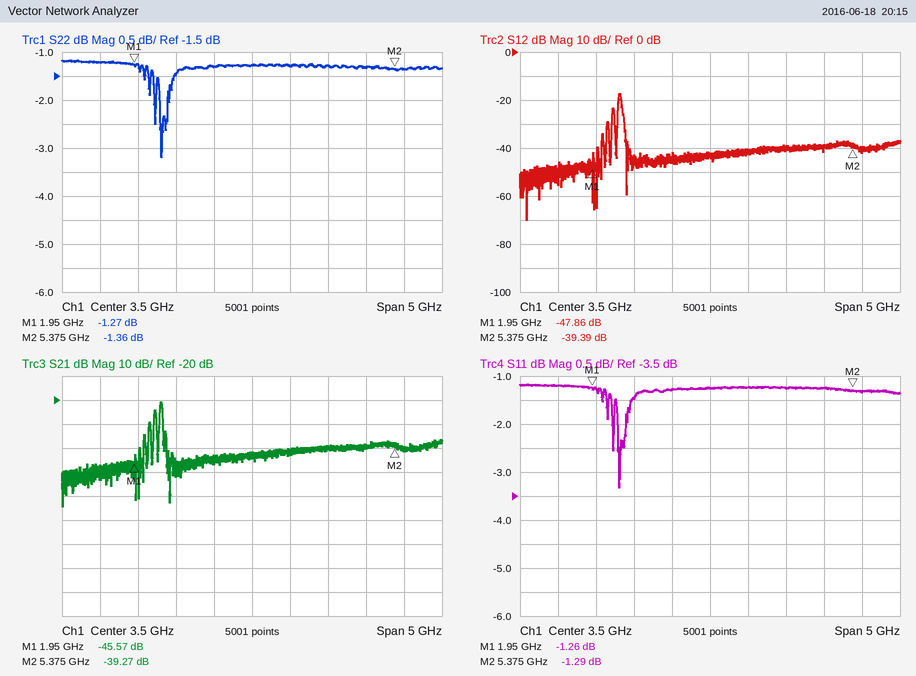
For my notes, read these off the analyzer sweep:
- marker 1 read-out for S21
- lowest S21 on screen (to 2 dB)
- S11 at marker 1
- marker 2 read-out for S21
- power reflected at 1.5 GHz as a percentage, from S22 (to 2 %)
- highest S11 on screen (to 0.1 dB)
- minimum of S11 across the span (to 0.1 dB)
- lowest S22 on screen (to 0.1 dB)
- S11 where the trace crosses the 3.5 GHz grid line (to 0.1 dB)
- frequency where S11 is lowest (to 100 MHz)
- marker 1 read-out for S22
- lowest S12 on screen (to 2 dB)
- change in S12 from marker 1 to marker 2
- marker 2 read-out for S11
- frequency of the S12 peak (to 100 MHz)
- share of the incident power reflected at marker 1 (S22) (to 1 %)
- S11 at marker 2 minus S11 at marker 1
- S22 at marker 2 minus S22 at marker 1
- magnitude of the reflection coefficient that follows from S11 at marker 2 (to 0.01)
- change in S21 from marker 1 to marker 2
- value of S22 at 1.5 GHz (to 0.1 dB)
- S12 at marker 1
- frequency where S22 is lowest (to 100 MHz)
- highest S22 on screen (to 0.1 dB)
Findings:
-45.57 dB
-64 dB
-1.26 dB
-39.27 dB
76 %
-1.2 dB
-3.3 dB
-3.2 dB
-1.2 dB
2.3 GHz
-1.27 dB
-70 dB
8.47 dB
-1.29 dB
2.3 GHz
75 %
-0.03 dB
-0.09 dB
0.86
6.30 dB
-1.2 dB
-47.86 dB
2.3 GHz
-1.2 dB
